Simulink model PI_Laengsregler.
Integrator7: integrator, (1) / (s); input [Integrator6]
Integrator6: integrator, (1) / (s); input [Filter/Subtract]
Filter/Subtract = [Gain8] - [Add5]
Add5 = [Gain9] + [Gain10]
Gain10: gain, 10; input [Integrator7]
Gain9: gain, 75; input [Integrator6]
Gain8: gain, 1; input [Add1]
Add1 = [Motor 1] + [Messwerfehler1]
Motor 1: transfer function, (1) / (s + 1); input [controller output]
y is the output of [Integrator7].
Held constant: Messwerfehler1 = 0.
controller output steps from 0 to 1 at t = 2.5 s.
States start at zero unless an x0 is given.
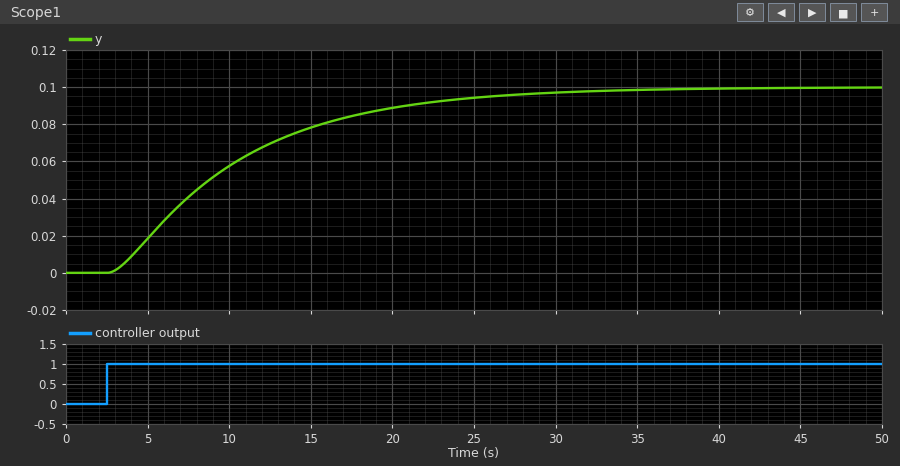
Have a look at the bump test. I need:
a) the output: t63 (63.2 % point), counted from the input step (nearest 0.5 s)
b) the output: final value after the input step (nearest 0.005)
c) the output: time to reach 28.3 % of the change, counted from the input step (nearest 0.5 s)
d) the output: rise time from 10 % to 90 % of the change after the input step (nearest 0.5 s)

8.5 s
0.100
3.5 s
16.5 s
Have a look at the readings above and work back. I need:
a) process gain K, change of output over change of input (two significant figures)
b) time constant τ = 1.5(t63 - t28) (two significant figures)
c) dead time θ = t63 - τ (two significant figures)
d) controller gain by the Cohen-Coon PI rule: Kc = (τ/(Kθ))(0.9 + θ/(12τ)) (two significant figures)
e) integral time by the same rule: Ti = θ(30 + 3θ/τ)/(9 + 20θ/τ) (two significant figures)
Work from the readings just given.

0.10
7.5 s
1.0 s
68
2.6 s
